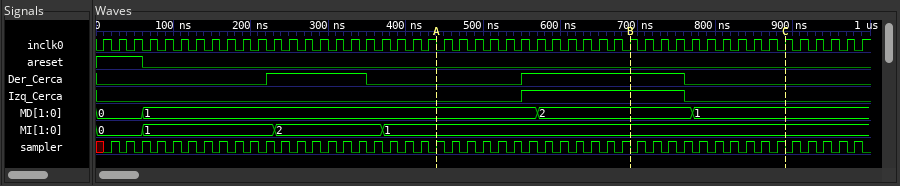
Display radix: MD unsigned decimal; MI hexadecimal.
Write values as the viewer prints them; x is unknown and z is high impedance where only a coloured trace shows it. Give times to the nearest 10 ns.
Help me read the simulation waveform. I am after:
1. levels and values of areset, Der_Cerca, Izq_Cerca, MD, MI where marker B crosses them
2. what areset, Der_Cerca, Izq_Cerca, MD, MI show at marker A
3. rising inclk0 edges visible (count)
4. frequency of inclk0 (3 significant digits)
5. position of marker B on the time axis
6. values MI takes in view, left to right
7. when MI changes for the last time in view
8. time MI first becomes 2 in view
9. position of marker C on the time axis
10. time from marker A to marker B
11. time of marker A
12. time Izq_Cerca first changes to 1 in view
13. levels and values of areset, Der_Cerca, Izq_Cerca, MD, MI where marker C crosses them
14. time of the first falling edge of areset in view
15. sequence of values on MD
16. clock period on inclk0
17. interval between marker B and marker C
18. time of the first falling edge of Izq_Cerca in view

areset=0, Der_Cerca=1, Izq_Cerca=1, MD=2, MI=1
areset=0, Der_Cerca=0, Izq_Cerca=0, MD=1, MI=1
50
50.0 MHz
690 ns
0, 1, 2, 1
370 ns
230 ns
890 ns
250 ns
440 ns
550 ns
areset=0, Der_Cerca=0, Izq_Cerca=0, MD=1, MI=1
60 ns
0, 1, 2, 1
20 ns
200 ns
760 ns
